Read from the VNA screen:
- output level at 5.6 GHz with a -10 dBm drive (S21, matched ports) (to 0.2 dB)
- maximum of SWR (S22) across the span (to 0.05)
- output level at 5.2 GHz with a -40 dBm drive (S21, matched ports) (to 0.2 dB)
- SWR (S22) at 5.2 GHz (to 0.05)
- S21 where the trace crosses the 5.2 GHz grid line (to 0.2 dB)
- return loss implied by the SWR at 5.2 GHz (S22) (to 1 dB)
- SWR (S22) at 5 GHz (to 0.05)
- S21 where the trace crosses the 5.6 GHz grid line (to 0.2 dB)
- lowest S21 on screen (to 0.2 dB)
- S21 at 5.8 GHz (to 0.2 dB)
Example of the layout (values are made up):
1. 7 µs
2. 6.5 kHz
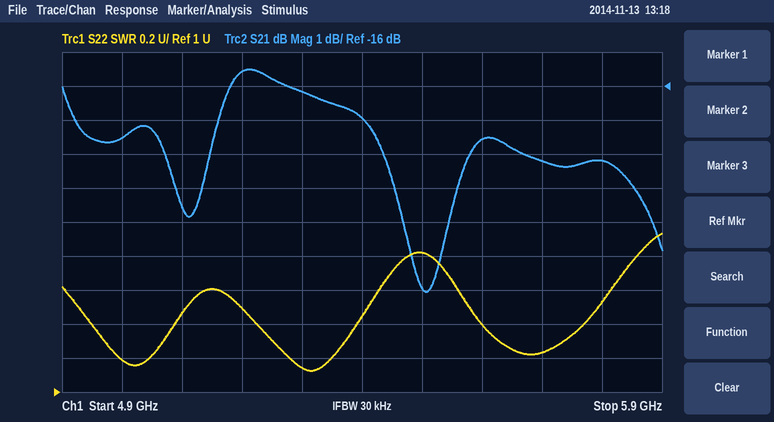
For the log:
1. -27.6 dBm
2. 1.95
3. -55.6 dBm
4. 1.50
5. -15.6 dB
6. 14 dB
7. 1.20
8. -17.6 dB
9. -22.0 dB
10. -18.2 dB
